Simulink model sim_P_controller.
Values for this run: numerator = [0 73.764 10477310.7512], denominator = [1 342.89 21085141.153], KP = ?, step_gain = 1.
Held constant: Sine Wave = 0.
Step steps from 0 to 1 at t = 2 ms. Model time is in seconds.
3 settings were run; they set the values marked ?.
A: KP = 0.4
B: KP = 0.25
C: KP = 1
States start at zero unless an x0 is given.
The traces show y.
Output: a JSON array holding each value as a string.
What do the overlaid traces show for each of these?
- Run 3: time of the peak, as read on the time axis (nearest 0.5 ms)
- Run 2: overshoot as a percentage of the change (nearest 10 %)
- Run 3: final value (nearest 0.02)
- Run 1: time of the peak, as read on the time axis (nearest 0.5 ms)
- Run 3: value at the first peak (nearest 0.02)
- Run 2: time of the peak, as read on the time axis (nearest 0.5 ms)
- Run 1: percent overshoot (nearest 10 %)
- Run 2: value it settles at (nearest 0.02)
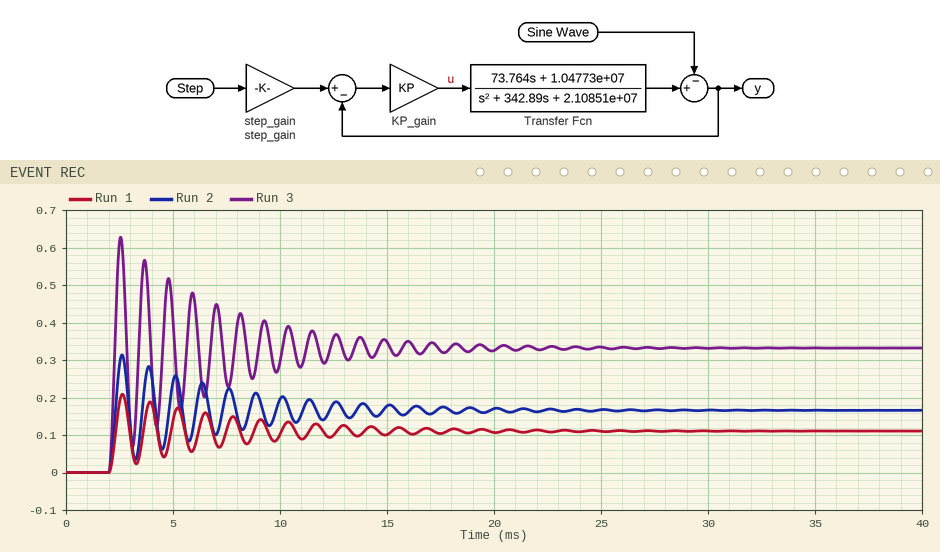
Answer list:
["2.5 ms", "90 %", "0.34", "2.5 ms", "0.62", "2.5 ms", "90 %", "0.16"]
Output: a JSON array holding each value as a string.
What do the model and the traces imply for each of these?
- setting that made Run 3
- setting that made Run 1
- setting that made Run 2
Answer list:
["C", "B", "A"]
